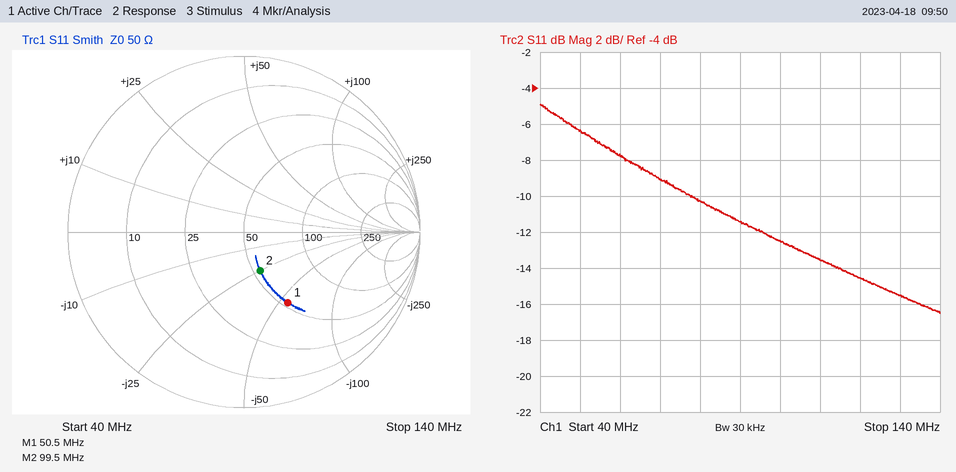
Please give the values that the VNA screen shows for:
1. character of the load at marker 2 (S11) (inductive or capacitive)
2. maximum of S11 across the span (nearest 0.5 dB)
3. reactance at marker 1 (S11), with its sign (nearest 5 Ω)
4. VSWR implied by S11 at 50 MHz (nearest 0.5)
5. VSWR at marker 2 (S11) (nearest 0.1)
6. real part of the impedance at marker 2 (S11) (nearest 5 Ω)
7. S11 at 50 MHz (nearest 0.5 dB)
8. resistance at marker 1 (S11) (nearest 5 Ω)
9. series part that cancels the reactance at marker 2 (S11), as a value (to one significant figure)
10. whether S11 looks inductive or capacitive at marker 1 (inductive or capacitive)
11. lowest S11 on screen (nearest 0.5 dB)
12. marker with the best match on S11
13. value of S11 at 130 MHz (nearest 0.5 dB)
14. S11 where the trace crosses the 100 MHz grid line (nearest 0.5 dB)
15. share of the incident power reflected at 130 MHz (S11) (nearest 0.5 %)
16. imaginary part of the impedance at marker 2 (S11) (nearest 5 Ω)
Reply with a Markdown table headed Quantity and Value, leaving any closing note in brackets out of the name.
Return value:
| Quantity | Value |
|---|---|
| character of the load at marker 2 (S11) | capacitive |
| maximum of S11 across the span | -5.0 dB |
| reactance at marker 1 (S11), with its sign | -55 Ω |
| VSWR implied by S11 at 50 MHz | 3.0 |
| VSWR at marker 2 (S11) | 1.6 |
| real part of the impedance at marker 2 (S11) | 55 Ω |
| S11 at 50 MHz | -6.5 dB |
| resistance at marker 1 (S11) | 55 Ω |
| series part that cancels the reactance at marker 2 (S11), as a value | 40 nH |
| whether S11 looks inductive or capacitive at marker 1 | capacitive |
| lowest S11 on screen | -16.5 dB |
| marker with the best match on S11 | marker 2 |
| value of S11 at 130 MHz | -15.5 dB |
| S11 where the trace crosses the 100 MHz grid line | -12.5 dB |
| share of the incident power reflected at 130 MHz (S11) | 3.0 % |
| imaginary part of the impedance at marker 2 (S11) | -25 Ω |
